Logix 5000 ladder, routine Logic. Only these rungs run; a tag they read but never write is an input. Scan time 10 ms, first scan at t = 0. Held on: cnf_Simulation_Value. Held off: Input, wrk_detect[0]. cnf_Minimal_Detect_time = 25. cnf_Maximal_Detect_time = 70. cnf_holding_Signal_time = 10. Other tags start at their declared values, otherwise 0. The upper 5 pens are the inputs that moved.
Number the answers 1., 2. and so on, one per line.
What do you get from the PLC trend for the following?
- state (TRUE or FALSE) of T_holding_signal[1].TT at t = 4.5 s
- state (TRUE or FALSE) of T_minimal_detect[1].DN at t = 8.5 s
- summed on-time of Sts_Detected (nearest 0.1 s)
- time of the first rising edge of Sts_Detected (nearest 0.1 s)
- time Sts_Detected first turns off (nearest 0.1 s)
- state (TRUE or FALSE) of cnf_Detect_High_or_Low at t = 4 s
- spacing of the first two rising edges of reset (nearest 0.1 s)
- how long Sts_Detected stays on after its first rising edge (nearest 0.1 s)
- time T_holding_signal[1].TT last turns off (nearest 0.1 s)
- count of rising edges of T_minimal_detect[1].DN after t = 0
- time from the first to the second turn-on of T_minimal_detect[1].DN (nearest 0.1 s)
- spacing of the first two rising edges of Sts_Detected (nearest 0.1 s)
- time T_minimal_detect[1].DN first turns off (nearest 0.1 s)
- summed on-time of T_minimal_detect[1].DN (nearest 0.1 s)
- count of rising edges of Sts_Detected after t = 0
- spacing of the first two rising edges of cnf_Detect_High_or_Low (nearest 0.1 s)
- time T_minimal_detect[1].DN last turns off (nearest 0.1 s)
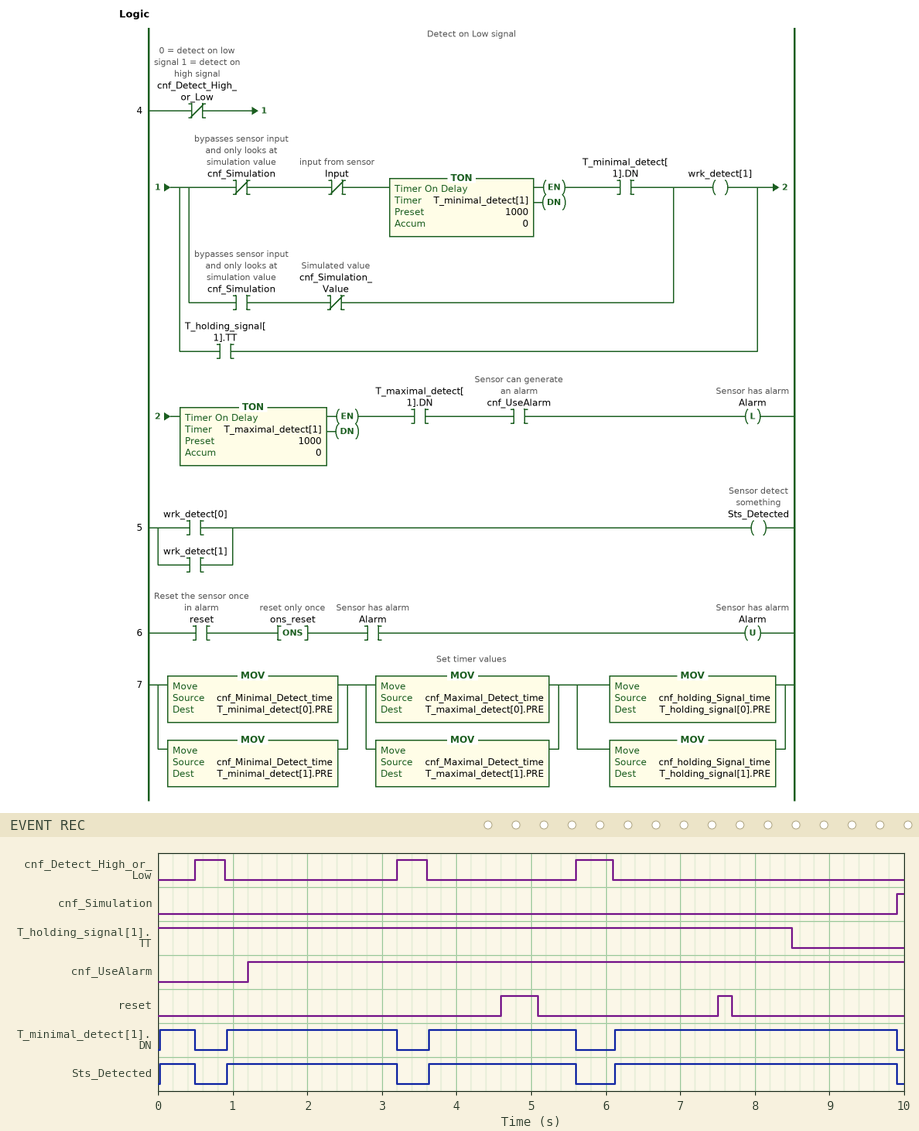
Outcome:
1. TRUE
2. TRUE
3. 8.5 s
4. 0.0 s
5. 0.5 s
6. FALSE
7. 2.9 s
8. 0.5 s
9. 8.5 s
10. 4
11. 0.9 s
12. 0.9 s
13. 0.5 s
14. 8.5 s
15. 4
16. 2.7 s
17. 9.9 s
